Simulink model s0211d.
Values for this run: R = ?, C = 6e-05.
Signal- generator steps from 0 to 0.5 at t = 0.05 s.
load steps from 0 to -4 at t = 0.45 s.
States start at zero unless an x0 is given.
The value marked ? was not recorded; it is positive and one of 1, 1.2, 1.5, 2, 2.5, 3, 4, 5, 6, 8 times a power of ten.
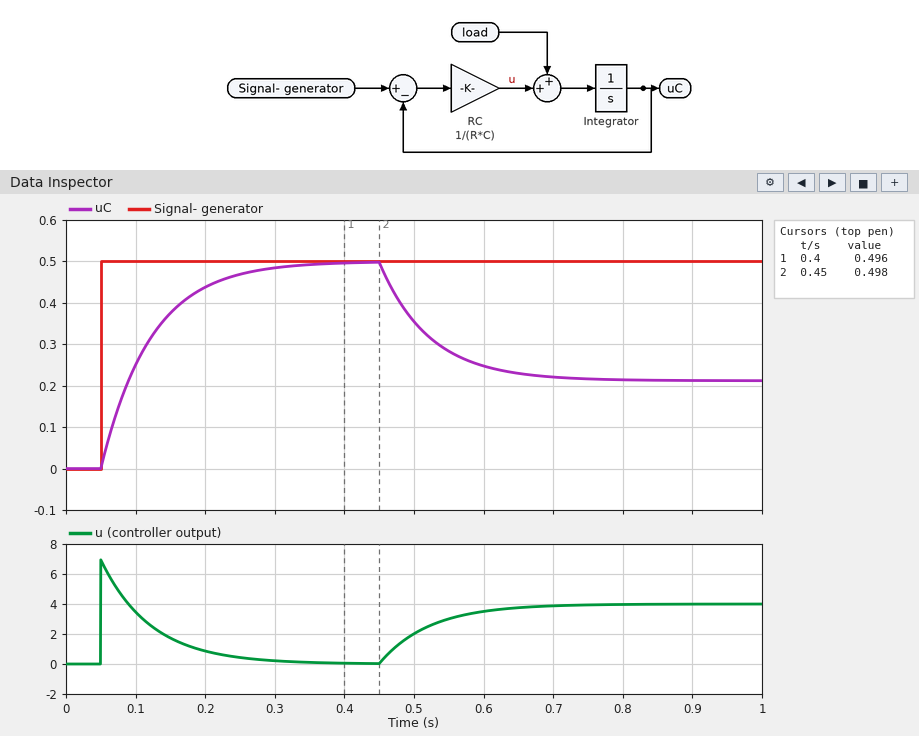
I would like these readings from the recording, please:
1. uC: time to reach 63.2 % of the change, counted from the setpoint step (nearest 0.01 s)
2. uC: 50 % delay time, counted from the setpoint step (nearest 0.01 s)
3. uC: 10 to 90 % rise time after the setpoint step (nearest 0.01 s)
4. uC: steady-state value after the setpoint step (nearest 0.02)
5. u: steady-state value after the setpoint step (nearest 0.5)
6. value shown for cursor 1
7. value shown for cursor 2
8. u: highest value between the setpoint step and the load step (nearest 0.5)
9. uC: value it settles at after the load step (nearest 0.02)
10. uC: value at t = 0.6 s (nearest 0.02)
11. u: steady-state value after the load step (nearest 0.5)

0.07 s
0.05 s
0.16 s
0.50
0.0
0.496
0.498
7.0
0.22
0.24
4.0
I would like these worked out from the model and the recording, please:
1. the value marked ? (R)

1200
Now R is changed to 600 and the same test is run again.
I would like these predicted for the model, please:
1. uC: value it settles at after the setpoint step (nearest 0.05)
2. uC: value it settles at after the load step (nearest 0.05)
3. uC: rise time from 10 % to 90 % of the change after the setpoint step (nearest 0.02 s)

0.50
0.35
0.08 s
